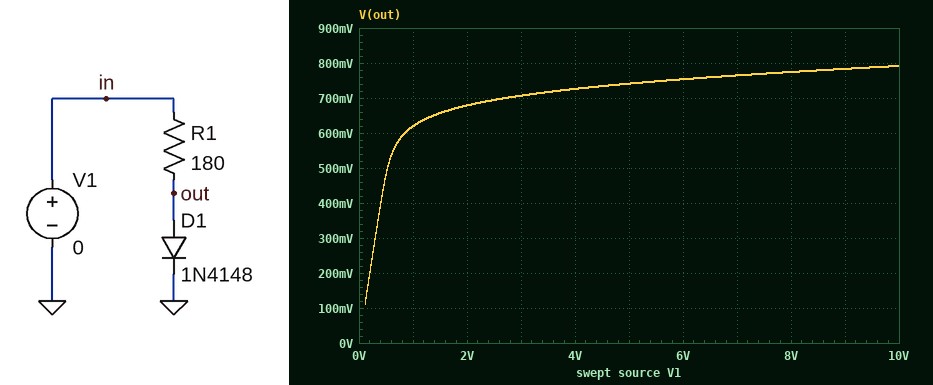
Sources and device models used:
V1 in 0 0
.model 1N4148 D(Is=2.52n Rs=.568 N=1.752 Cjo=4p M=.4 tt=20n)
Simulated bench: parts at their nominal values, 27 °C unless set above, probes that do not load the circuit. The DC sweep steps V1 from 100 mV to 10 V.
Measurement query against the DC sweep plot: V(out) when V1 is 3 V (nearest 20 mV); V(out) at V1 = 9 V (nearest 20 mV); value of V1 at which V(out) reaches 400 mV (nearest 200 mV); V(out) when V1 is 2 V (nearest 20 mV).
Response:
700 mV
780 mV
400 mV
680 mV
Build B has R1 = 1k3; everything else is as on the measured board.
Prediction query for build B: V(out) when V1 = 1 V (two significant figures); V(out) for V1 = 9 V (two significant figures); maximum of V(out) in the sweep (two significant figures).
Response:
540 mV
670 mV
680 mV
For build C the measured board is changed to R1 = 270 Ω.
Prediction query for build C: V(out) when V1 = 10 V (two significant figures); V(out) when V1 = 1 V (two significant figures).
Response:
760 mV
600 mV
